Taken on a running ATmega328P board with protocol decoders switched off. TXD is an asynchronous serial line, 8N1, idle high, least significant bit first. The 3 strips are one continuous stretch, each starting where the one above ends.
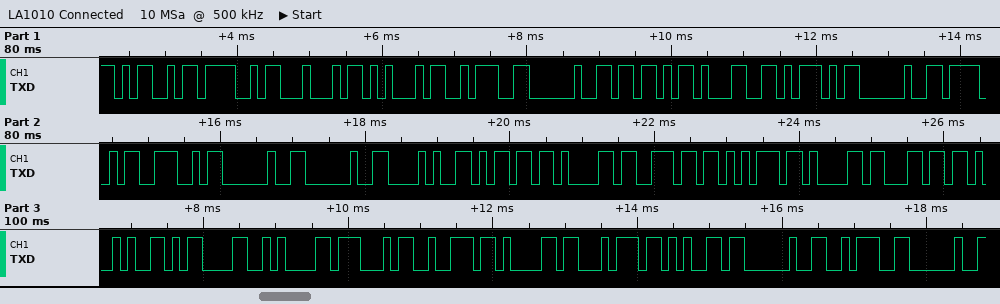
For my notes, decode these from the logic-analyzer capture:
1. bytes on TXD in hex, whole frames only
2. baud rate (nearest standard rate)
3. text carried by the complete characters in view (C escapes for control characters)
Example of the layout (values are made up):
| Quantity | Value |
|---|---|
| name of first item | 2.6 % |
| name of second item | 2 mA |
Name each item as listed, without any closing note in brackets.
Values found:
| Quantity | Value |
|---|---|
| bytes on TXD in hex, whole frames only | 4D 4F 44 45 3A 20 5B 31 5D 20 4F 4E 20 20 28 6D 61 6E 75 61 6C 29 0D 0A 47 72 61 74 65 20 3A 20 |
| baud rate | 9600 baud |
| text carried by the complete characters in view | "MODE: [1] ON  (manual)\r\nGrate : " |
